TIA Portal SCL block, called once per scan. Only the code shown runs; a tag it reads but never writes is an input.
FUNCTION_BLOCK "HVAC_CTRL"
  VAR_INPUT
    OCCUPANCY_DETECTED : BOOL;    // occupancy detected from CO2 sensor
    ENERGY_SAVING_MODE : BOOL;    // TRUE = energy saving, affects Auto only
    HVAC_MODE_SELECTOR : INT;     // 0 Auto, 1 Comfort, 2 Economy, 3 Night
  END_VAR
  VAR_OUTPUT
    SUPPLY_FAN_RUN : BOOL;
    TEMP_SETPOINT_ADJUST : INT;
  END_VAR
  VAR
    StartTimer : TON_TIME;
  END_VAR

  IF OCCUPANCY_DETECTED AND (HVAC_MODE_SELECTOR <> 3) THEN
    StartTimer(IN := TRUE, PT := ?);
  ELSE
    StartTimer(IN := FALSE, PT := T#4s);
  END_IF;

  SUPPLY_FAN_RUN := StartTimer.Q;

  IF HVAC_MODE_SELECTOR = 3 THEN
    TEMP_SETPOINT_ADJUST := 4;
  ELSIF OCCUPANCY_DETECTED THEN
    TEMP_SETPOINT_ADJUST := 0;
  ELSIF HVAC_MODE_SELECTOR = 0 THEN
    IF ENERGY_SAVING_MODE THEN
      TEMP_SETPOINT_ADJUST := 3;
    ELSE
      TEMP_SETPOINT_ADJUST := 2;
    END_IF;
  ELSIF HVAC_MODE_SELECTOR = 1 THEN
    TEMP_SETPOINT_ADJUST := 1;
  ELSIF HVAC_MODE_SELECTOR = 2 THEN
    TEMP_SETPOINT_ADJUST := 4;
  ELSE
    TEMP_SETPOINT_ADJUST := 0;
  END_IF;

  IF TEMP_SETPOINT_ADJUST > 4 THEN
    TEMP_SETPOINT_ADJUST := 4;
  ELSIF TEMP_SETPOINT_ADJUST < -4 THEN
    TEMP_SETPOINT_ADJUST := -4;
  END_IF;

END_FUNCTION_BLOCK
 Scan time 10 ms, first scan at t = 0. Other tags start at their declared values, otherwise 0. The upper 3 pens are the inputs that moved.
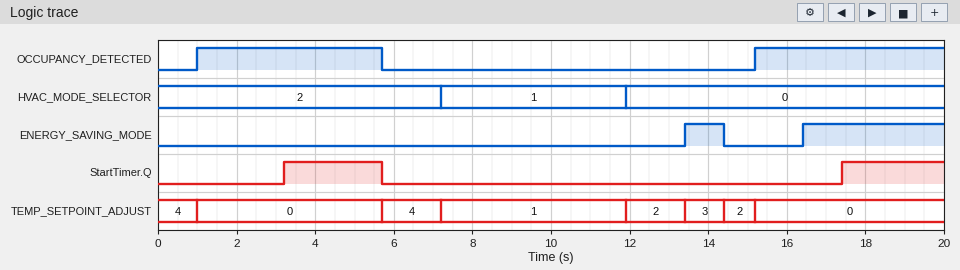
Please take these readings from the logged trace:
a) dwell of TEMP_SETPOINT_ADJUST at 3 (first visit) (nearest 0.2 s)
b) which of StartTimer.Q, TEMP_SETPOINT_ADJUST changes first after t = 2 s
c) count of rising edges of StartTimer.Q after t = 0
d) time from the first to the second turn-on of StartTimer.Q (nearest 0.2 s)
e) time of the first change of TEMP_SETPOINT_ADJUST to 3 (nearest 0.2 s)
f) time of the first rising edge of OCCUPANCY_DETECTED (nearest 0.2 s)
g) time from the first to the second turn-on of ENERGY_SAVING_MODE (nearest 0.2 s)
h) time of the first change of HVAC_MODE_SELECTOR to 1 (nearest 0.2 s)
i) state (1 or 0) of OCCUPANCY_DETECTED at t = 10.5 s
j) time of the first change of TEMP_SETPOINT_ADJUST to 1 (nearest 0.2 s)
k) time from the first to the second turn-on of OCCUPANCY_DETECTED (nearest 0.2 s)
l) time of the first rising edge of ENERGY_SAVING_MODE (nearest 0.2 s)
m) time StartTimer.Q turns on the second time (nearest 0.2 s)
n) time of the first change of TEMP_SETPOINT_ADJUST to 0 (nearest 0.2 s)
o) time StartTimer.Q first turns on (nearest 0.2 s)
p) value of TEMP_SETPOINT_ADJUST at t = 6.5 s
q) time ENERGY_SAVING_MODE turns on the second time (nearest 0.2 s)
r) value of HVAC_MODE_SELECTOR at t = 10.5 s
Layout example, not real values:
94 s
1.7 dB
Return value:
1.0 s
StartTimer.Q
2
14.2 s
13.4 s
1.0 s
3.0 s
7.2 s
0
7.2 s
14.2 s
13.4 s
17.4 s
1.0 s
3.2 s
4
16.4 s
1
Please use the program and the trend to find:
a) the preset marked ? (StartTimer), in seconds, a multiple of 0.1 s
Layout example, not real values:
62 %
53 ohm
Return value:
2.2 s
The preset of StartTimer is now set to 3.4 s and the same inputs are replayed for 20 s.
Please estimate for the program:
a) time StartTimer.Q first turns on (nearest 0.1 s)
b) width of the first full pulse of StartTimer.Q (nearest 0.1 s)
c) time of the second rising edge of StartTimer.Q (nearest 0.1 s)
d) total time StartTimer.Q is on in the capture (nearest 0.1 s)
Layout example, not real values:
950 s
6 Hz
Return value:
4.4 s
1.3 s
18.6 s
2.7 s
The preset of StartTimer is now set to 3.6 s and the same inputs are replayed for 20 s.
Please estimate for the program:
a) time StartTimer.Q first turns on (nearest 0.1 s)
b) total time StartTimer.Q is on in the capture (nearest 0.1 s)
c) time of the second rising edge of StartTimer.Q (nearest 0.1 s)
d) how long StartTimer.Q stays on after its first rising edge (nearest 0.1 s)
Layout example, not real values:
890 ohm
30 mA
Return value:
4.6 s
2.3 s
18.8 s
1.1 s
